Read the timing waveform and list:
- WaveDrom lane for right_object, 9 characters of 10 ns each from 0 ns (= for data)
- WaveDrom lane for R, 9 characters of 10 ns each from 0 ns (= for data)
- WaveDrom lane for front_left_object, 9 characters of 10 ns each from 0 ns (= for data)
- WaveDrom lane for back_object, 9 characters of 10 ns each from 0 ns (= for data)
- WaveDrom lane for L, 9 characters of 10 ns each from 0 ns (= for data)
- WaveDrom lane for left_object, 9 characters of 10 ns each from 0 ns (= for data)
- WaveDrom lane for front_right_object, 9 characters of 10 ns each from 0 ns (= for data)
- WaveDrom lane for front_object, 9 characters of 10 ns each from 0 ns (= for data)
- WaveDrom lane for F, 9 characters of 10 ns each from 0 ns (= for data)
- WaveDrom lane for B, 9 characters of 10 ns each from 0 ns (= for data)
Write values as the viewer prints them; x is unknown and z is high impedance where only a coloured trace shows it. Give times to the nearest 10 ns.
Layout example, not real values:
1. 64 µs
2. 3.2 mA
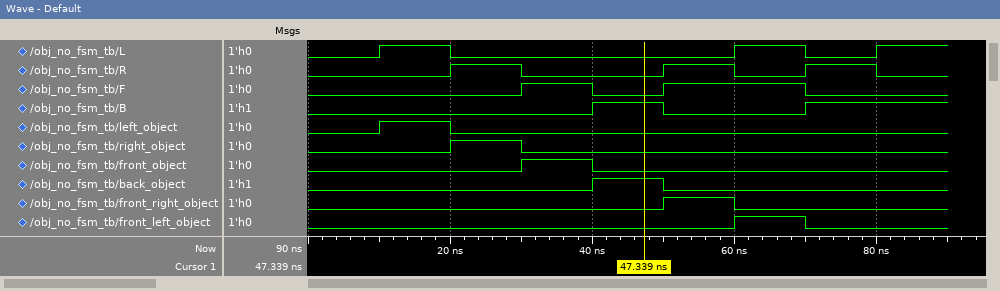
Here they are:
1. {name: 'right_object', wave: '0.10.....'}
2. {name: 'R', wave: '0.10.1010'}
3. {name: 'front_left_object', wave: '0.....10.'}
4. {name: 'back_object', wave: '0...10...'}
5. {name: 'L', wave: '010...101'}
6. {name: 'left_object', wave: '010......'}
7. {name: 'front_right_object', wave: '0....10..'}
8. {name: 'front_object', wave: '0..10....'}
9. {name: 'F', wave: '0..101.0.'}
10. {name: 'B', wave: '0...10.1.'}
